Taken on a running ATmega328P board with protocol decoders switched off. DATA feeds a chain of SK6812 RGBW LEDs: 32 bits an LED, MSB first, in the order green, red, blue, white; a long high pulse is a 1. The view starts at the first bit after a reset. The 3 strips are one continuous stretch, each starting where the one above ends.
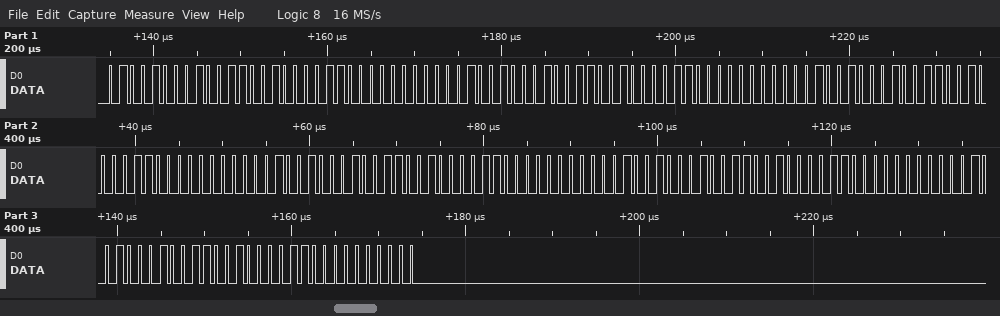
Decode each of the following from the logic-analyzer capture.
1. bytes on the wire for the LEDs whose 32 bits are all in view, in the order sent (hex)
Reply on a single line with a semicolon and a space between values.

48 99 0C 00 48 99 0C 00 48 99 0C 00 48 99 0C 00 48 99 0C 00 48 99 0C 00
